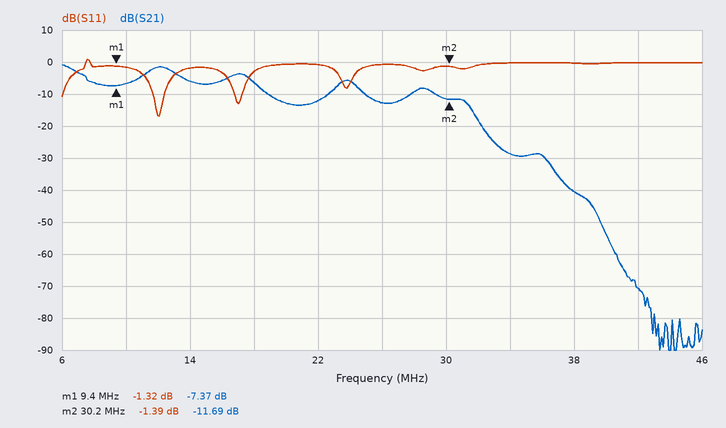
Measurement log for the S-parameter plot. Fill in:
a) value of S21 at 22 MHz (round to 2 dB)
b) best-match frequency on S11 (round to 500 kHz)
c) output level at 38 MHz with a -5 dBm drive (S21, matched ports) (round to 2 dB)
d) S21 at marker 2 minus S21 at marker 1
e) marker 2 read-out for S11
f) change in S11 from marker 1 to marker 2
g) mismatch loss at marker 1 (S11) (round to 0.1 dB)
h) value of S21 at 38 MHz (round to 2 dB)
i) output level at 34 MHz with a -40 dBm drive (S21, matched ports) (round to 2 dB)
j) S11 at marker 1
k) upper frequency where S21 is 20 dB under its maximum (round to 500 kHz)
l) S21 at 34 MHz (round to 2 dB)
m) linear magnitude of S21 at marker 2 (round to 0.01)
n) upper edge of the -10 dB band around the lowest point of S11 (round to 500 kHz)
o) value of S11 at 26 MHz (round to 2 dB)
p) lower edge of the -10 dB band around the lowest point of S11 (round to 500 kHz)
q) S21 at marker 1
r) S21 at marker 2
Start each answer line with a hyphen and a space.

- -12 dB
- 12.0 MHz
- -46 dBm
- -4.32 dB
- -1.39 dB
- -0.07 dB
- 5.8 dB
- -40 dB
- -68 dBm
- -1.32 dB
- 32.5 MHz
- -28 dB
- 0.26
- 12.5 MHz
- 0 dB
- 11.5 MHz
- -7.37 dB
- -11.69 dB
